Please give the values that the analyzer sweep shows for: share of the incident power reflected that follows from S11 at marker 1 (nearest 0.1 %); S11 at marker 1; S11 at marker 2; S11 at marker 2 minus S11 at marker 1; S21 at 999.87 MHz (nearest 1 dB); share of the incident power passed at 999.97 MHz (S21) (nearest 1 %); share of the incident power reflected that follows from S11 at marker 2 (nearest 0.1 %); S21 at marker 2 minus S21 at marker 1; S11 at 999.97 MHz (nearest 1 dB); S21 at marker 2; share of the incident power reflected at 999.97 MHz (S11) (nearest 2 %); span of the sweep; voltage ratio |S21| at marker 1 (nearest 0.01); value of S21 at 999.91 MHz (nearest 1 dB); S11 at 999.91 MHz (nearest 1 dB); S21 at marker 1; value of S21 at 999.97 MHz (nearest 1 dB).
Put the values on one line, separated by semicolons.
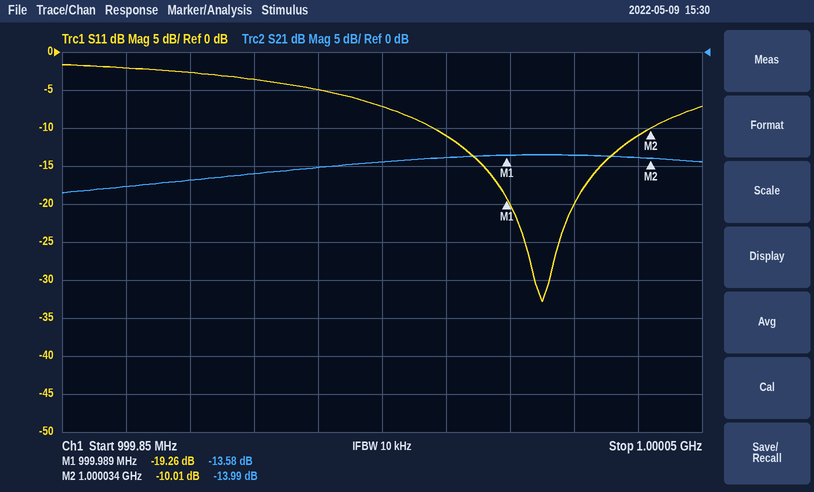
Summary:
1.2 %; -19.26 dB; -10.01 dB; 9.25 dB; -18 dB; 4 %; 10.0 %; -0.41 dB; -11 dB; -13.99 dB; 8 %; 200 kHz; 0.21; -16 dB; -4 dB; -13.58 dB; -14 dB
